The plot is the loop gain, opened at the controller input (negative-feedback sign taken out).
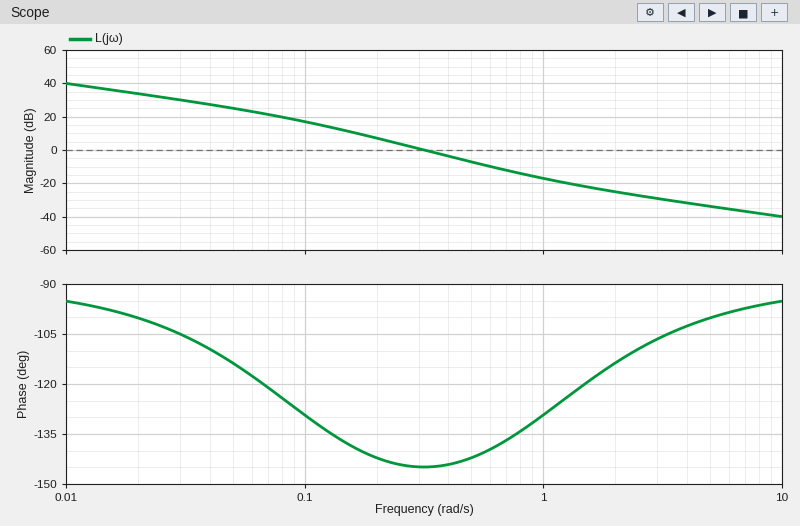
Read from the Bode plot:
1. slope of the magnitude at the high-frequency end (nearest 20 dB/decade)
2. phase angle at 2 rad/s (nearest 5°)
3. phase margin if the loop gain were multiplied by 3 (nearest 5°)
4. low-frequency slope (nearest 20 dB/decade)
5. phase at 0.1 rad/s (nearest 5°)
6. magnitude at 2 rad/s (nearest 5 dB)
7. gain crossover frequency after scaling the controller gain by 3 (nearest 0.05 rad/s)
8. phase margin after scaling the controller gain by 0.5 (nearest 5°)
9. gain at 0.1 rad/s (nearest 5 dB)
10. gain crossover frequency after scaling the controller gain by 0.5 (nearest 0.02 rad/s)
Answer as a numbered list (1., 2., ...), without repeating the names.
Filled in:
1. -20 dB/decade
2. -115°
3. 40°
4. -20 dB/decade
5. -130°
6. -25 dB
7. 0.60 rad/s
8. 35°
9. 15 dB
10. 0.22 rad/s
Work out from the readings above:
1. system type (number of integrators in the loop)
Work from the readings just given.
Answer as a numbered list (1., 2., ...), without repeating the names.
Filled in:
1. 1
